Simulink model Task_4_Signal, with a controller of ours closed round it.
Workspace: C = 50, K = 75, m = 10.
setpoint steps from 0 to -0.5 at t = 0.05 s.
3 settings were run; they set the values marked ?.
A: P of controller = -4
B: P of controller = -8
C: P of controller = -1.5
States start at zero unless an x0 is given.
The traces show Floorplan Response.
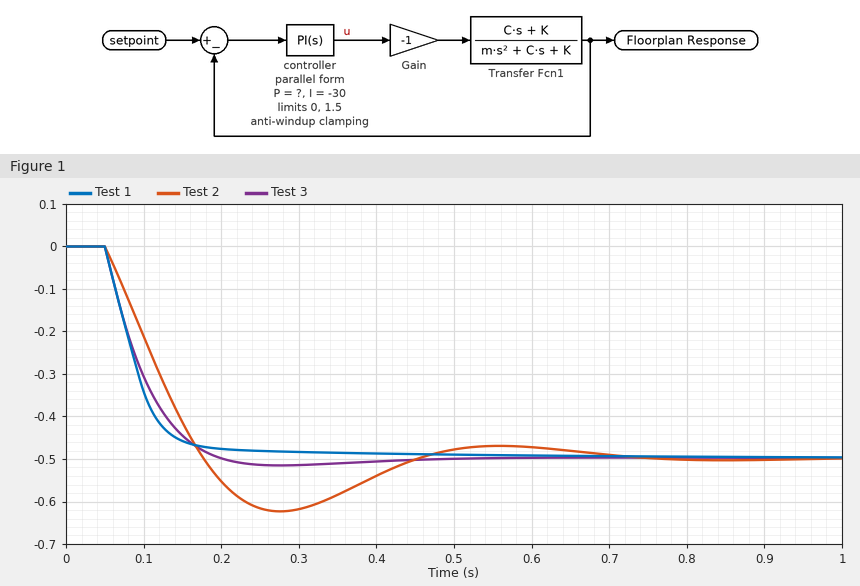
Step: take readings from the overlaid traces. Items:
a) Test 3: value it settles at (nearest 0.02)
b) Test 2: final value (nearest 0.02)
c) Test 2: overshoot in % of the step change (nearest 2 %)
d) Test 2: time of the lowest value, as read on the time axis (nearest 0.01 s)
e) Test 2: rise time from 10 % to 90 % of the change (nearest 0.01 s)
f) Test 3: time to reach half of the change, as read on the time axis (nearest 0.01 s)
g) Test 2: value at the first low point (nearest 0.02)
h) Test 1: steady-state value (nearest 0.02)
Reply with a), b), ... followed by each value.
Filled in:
a) -0.50
b) -0.50
c) 24 %
d) 0.28 s
e) 0.10 s
f) 0.09 s
g) -0.62
h) -0.50
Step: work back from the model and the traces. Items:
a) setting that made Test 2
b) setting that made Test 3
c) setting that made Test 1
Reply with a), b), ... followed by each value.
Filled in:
a) C
b) A
c) B
